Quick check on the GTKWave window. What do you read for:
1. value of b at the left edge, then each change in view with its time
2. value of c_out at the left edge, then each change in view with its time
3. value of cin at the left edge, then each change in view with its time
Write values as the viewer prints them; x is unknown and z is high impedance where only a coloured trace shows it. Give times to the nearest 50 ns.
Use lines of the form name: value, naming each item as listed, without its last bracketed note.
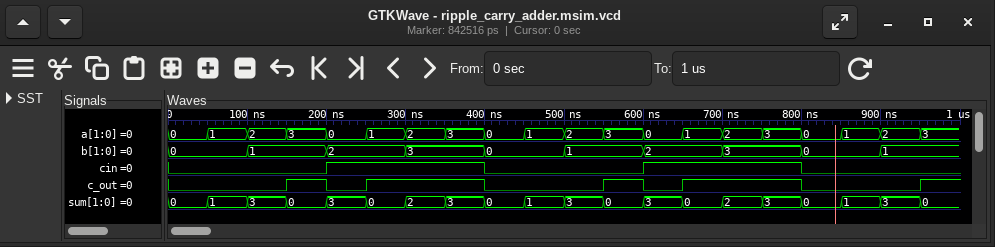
value of b at the left edge, then each change in view with its time: 0, 1 at 100 ns, 2 at 200 ns, 3 at 300 ns, 0 at 400 ns, 1 at 500 ns, 2 at 600 ns, 3 at 700 ns, 0 at 800 ns, 1 at 900 ns
value of c_out at the left edge, then each change in view with its time: 0, 1 at 150 ns, 0 at 200 ns, 1 at 250 ns, 0 at 400 ns, 1 at 550 ns, 0 at 600 ns, 1 at 650 ns, 0 at 800 ns, 1 at 950 ns
value of cin at the left edge, then each change in view with its time: 0, 1 at 200 ns, 0 at 400 ns, 1 at 600 ns, 0 at 800 ns
